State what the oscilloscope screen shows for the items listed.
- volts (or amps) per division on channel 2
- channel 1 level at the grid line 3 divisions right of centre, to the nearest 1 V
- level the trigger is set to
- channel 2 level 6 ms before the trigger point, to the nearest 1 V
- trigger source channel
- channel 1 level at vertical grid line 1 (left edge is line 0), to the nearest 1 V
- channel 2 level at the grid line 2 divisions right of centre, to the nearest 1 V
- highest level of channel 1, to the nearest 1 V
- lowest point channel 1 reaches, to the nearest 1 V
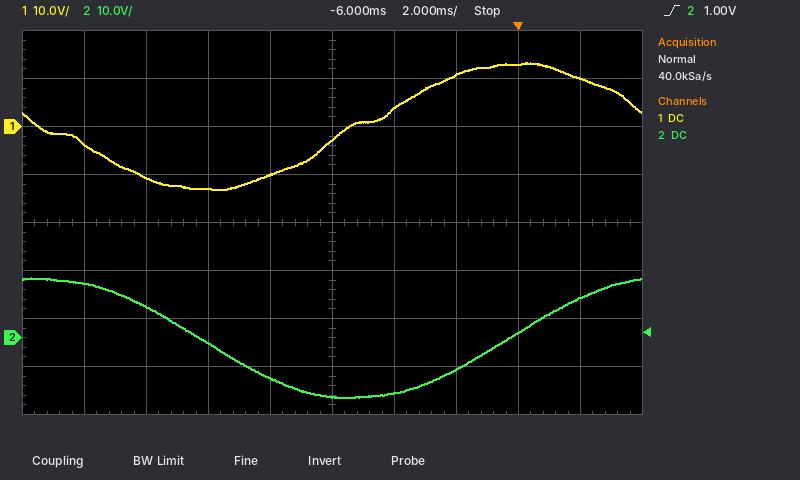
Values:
10 V
13 V
1.00 V
-12 V
channel 2
-4 V
-7 V
13 V
-13 V
